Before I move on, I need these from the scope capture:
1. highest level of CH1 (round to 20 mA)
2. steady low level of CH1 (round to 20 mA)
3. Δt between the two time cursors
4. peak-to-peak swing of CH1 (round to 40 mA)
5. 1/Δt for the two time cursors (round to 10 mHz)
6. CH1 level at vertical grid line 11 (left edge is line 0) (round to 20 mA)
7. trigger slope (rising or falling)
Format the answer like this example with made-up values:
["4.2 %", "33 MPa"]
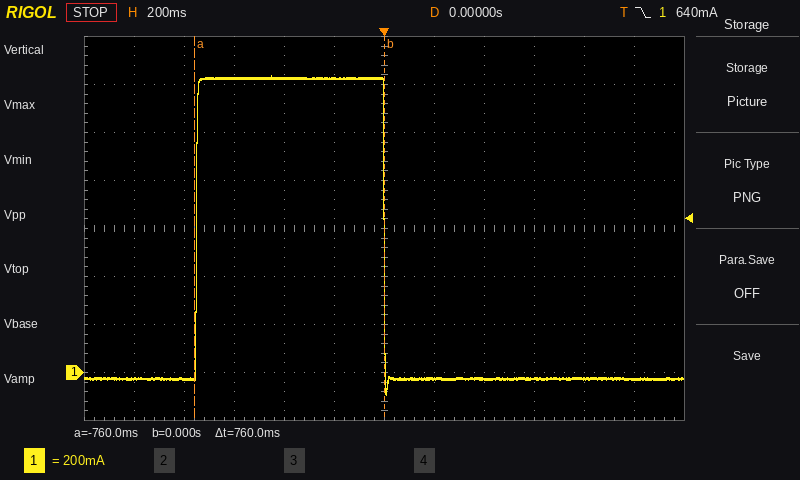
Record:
["1.24 A", "-20 mA", "760 ms", "1.32 A", "1.32 Hz", "-20 mA", "falling"]
